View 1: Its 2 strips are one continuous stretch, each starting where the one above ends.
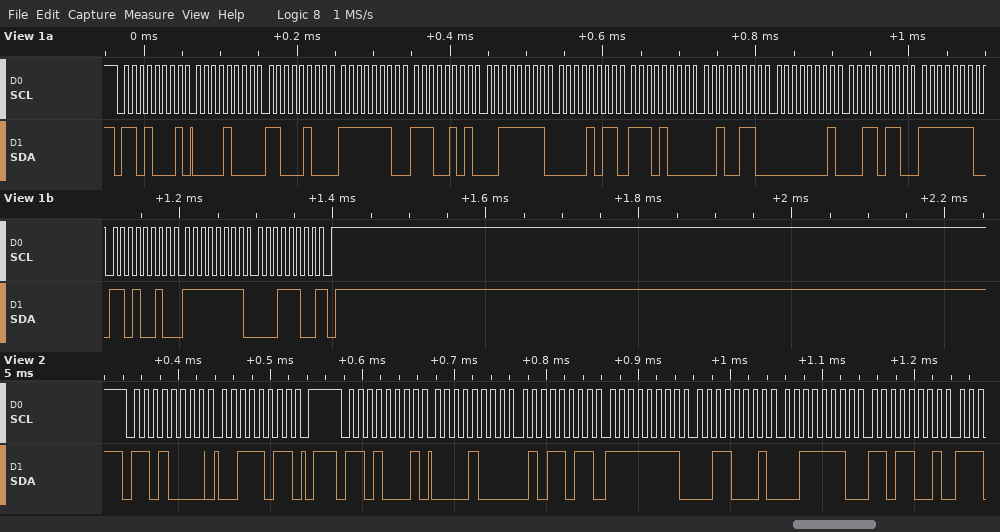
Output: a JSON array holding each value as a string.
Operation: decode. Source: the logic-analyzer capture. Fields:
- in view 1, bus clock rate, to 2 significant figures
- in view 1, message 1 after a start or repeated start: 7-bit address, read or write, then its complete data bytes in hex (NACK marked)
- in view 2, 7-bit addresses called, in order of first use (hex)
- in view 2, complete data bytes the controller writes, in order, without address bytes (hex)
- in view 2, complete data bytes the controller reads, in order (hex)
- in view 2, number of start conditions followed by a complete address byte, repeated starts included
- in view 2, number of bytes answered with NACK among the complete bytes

["100 kHz", "0x68 read: 08 C4 FE E5 3F 0B E8 26 01 36 FE D2 FF 1C NACK", "0x68", "3B", "08 5B FF 31 3E D9", "2", "0"]
